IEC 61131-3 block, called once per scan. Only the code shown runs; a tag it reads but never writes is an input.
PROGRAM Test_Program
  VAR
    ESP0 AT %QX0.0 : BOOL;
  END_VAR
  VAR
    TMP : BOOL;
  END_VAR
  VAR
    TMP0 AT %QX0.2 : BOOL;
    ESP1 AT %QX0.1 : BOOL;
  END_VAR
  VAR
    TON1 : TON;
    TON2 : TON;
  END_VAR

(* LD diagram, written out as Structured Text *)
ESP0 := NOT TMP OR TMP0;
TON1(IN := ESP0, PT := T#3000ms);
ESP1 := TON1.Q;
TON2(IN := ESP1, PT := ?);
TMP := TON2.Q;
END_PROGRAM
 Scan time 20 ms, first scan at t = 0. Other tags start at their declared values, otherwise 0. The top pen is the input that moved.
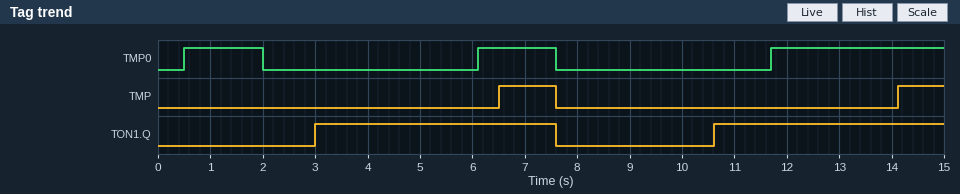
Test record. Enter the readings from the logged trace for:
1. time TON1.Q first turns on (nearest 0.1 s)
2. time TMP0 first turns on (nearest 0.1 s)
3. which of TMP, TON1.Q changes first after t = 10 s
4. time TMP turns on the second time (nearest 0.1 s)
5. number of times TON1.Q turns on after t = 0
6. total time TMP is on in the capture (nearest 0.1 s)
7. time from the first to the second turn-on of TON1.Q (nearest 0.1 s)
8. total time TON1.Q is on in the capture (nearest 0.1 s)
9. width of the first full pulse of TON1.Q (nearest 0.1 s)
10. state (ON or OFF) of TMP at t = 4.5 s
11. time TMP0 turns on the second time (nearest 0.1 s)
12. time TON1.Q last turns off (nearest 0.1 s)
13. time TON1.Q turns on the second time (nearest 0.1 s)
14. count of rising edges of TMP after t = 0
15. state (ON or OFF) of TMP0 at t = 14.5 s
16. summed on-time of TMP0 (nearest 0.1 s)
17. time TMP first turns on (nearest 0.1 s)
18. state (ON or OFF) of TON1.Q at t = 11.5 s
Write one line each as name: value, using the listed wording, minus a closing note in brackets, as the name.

time TON1.Q first turns on: 3.0 s
time TMP0 first turns on: 0.5 s
which of TMP, TON1.Q changes first after t = 10 s: TON1.Q
time TMP turns on the second time: 14.1 s
number of times TON1.Q turns on after t = 0: 2
total time TMP is on in the capture: 2.0 s
time from the first to the second turn-on of TON1.Q: 7.6 s
total time TON1.Q is on in the capture: 9.0 s
width of the first full pulse of TON1.Q: 4.6 s
state (ON or OFF) of TMP at t = 4.5 s: OFF
time TMP0 turns on the second time: 6.1 s
time TON1.Q last turns off: 7.6 s
time TON1.Q turns on the second time: 10.6 s
count of rising edges of TMP after t = 0: 2
state (ON or OFF) of TMP0 at t = 14.5 s: ON
summed on-time of TMP0: 6.3 s
time TMP first turns on: 6.5 s
state (ON or OFF) of TON1.Q at t = 11.5 s: ON
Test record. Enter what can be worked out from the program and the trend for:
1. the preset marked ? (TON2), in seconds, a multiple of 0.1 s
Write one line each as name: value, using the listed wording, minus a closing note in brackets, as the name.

the preset marked ? (TON2), in seconds, a multiple of 0.1 s: 3.5 s
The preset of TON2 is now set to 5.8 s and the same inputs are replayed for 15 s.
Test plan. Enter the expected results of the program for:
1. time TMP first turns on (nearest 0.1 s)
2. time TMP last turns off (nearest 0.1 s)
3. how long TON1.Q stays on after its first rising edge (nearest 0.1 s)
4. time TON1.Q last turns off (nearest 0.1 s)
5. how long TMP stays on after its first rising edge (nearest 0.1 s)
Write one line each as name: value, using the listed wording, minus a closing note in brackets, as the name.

time TMP first turns on: 8.8 s
time TMP last turns off: 8.8 s
how long TON1.Q stays on after its first rising edge: 5.8 s
time TON1.Q last turns off: 8.8 s
how long TMP stays on after its first rising edge: 0.0 s
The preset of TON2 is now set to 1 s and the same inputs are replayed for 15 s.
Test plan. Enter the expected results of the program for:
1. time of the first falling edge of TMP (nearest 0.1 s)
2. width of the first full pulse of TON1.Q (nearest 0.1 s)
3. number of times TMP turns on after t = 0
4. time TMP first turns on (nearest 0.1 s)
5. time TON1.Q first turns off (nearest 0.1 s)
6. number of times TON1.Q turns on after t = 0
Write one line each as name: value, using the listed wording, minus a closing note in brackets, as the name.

time of the first falling edge of TMP: 4.0 s
width of the first full pulse of TON1.Q: 1.0 s
number of times TMP turns on after t = 0: 3
time TMP first turns on: 4.0 s
time TON1.Q first turns off: 4.0 s
number of times TON1.Q turns on after t = 0: 3
